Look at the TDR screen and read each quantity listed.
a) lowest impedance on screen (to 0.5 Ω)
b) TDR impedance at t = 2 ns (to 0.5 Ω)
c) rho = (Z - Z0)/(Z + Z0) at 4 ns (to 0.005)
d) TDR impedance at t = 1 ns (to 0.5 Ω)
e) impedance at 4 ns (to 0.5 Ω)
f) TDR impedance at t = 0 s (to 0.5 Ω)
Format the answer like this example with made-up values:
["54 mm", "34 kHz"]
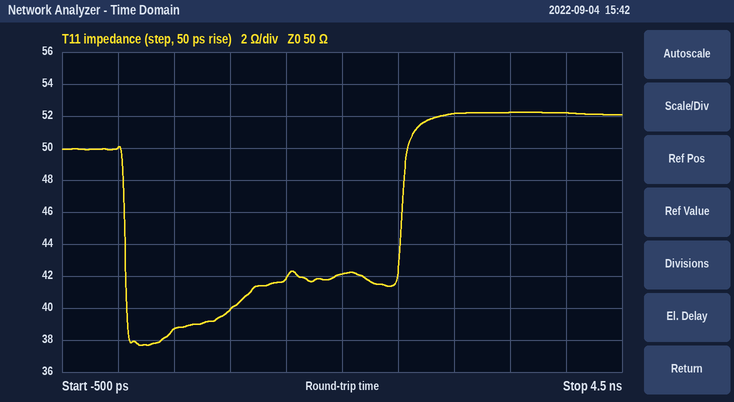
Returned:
["37.5 Ω", "42.0 Ω", "+0.020", "40.0 Ω", "52.0 Ω", "50.0 Ω"]
